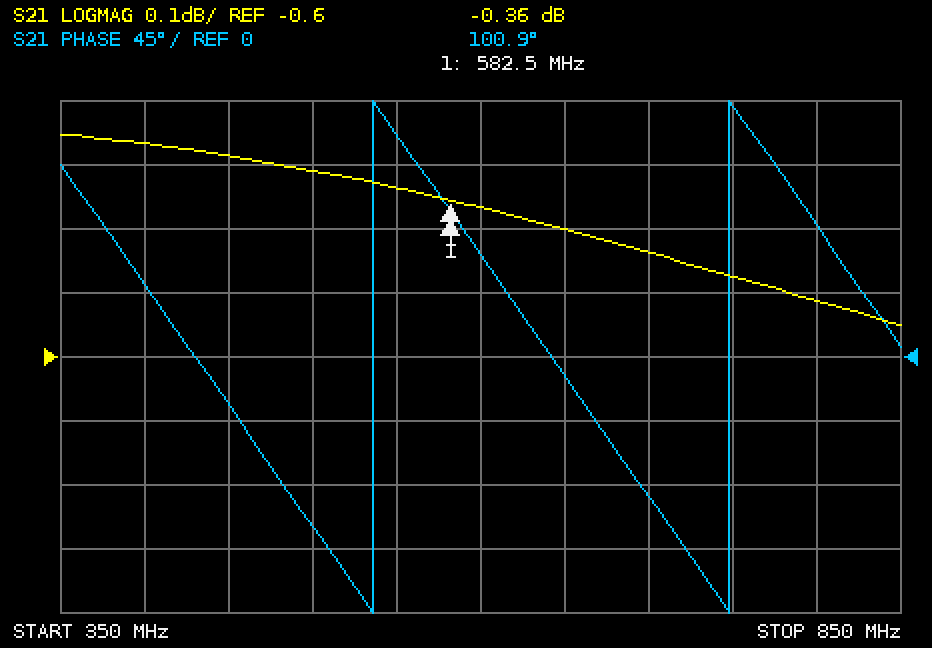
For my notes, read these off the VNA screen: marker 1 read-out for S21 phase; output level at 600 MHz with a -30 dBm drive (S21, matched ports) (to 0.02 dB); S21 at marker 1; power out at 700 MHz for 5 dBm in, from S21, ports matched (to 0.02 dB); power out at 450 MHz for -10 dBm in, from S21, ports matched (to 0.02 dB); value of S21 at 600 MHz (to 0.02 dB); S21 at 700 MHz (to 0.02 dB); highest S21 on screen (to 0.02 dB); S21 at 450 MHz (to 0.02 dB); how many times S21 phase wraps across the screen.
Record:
100.9°
-30.36 dBm
-0.36 dB
4.56 dBm
-10.28 dBm
-0.36 dB
-0.44 dB
-0.26 dB
-0.28 dB
2
